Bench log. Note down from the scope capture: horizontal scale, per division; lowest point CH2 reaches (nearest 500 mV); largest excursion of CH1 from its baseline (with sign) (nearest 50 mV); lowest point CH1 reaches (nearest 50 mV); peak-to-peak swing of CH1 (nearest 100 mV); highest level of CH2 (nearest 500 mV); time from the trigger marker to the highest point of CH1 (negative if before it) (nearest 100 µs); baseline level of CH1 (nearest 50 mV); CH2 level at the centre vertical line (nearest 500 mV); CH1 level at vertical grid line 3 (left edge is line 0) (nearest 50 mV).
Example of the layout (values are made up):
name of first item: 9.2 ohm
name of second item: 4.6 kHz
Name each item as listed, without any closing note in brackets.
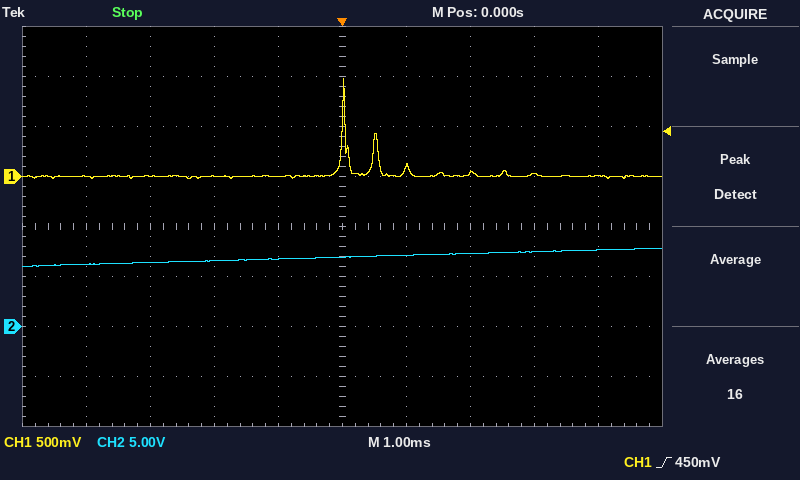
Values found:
horizontal scale, per division: 1 ms
lowest point CH2 reaches: 6.0 V
largest excursion of CH1 from its baseline (with sign): +1.00 V
lowest point CH1 reaches: 0 mV
peak-to-peak swing of CH1: 1.00 V
highest level of CH2: 8.0 V
time from the trigger marker to the highest point of CH1 (negative if before it): 0.0 ms
baseline level of CH1: 0 mV
CH2 level at the centre vertical line: 7.0 V
CH1 level at vertical grid line 3 (left edge is line 0): 0 mV
